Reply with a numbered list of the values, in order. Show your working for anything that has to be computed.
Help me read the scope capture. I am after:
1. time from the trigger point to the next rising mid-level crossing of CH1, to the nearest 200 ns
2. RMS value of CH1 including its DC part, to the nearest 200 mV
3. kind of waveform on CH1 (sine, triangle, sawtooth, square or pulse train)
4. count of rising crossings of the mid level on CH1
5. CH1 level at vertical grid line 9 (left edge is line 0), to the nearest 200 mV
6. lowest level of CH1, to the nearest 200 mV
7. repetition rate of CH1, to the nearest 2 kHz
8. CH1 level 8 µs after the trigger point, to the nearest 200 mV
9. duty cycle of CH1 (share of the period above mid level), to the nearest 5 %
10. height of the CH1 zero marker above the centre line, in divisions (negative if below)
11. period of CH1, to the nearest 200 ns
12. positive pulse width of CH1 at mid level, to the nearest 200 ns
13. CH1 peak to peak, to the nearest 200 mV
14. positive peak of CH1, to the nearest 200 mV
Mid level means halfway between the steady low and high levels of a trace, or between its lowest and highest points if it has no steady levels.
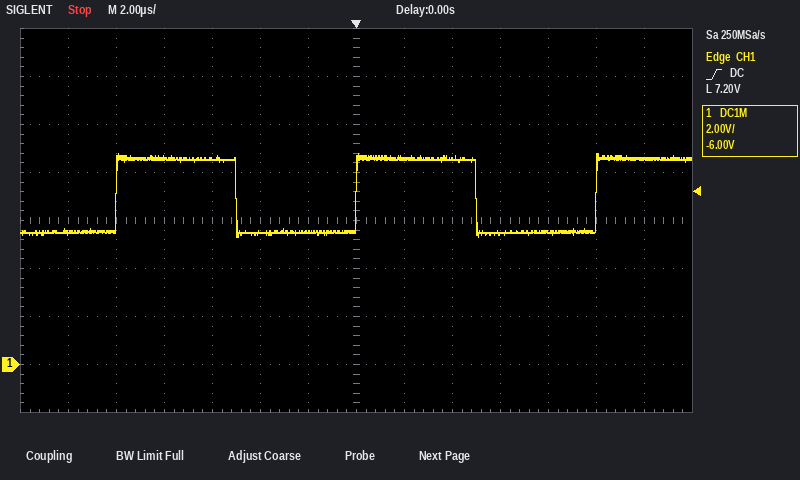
1. 10.0 µs
2. √(0.5 × (8.8 V)² + 0.5 × (5.2 V)²) ≈ 7.2 V
3. square
4. 3
5. 8.6 V
6. 5.2 V
7. 1 / 10.0 µs ≈ 100 kHz
8. 5.6 V
9. 5.0 µs / 10.0 µs ≈ 50 %
10. -3.0 div
11. 10.0 µs
12. 5.0 µs
13. 8.8 V − (5.2 V) = 3.6 V
14. 8.8 V
